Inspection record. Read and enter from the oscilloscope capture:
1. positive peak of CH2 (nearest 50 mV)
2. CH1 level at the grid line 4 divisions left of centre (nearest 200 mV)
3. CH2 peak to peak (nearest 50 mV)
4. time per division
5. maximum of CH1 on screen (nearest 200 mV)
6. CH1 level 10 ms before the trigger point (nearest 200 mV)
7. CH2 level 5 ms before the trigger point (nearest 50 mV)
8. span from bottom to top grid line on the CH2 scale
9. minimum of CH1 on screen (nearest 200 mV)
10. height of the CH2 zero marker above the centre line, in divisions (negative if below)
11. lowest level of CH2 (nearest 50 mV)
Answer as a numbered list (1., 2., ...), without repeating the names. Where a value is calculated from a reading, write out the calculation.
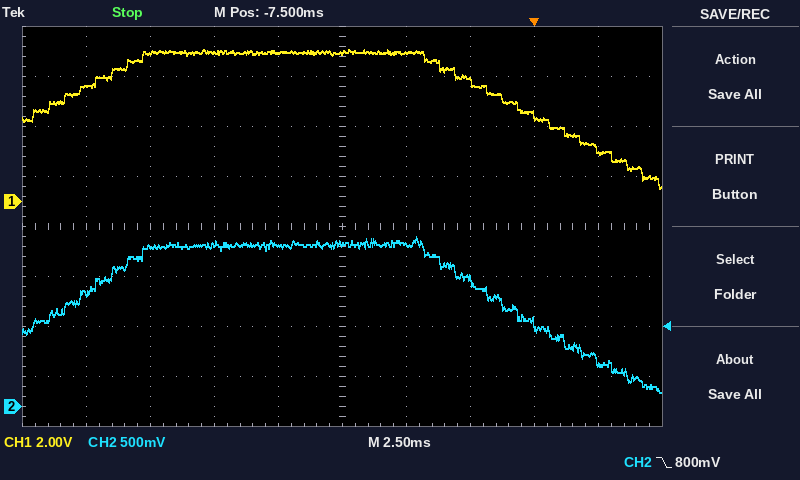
1. 1.70 V
2. 4.6 V
3. 1.70 V − (150 mV) = 1.55 V
4. 2.5 ms
5. 6.0 V
6. 6.0 V
7. 1.60 V
8. 4 V
9. 600 mV
10. -3.6 div
11. 150 mV
